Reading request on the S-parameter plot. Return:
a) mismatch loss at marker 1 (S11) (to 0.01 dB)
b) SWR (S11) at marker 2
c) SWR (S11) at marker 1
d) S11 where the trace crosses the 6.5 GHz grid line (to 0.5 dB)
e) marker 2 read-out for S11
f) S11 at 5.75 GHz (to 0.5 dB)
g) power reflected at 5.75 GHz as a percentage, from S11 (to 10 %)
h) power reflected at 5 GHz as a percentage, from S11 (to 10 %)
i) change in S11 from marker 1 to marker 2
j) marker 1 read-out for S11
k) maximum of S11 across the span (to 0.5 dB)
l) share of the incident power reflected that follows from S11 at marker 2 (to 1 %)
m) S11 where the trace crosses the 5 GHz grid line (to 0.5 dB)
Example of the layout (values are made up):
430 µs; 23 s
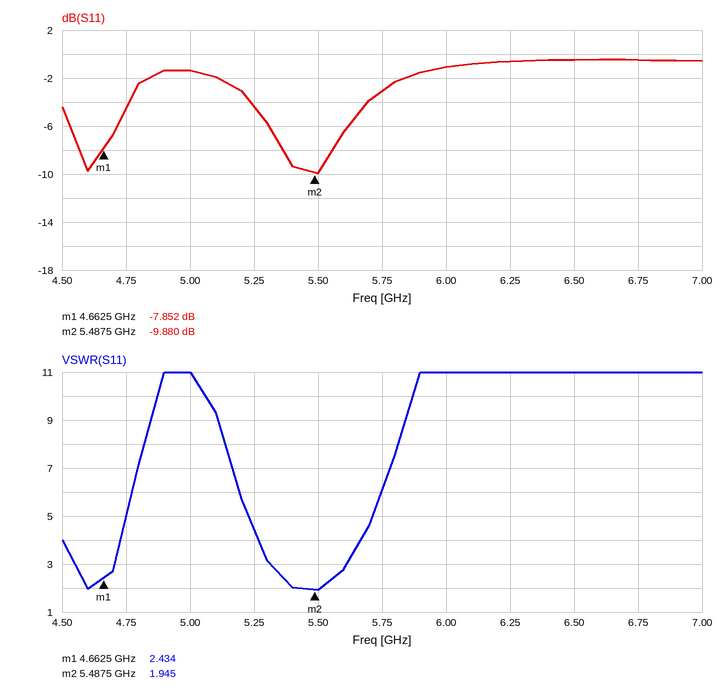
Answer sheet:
0.78 dB; 1.945; 2.434; -0.5 dB; -9.880 dB; -3.0 dB; 50 %; 70 %; -2.028 dB; -7.852 dB; -0.5 dB; 10 %; -1.5 dB
